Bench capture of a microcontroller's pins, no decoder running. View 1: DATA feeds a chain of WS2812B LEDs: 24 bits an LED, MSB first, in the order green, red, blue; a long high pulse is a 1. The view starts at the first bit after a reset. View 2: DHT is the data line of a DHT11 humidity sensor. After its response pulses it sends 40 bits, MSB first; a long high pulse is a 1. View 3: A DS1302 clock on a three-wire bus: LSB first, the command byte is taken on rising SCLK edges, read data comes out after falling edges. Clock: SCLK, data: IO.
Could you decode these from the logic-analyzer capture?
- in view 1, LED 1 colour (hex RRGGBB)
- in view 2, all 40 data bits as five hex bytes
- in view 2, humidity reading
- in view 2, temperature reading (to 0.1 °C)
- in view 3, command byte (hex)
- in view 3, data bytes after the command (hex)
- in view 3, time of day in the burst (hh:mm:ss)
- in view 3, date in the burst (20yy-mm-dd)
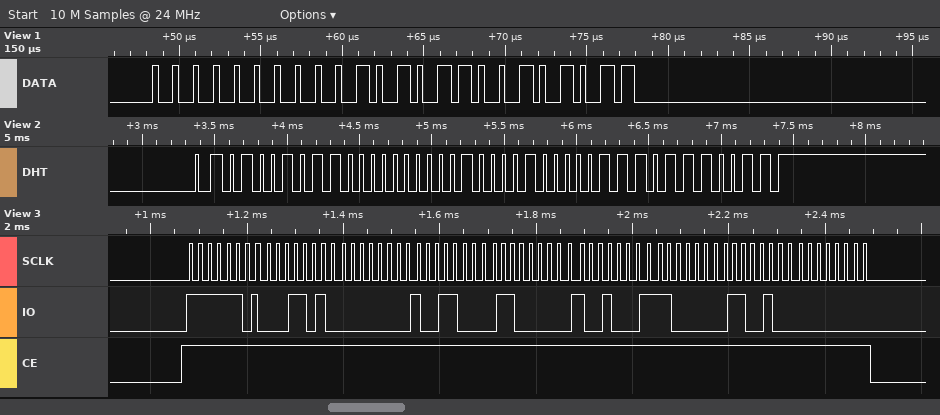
#2B002B
4B 00 21 07 73
75 %
33.7 °C
0xBF
58 00 19 06 12 07 26 00
19:00:58
2026-12-06
